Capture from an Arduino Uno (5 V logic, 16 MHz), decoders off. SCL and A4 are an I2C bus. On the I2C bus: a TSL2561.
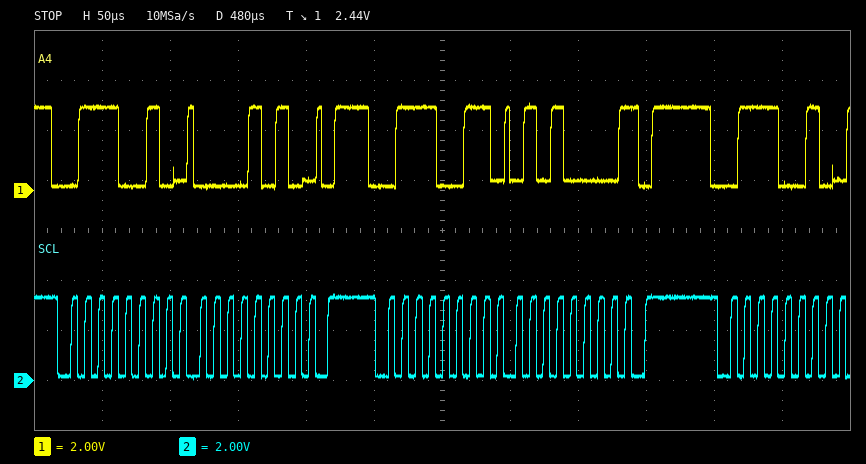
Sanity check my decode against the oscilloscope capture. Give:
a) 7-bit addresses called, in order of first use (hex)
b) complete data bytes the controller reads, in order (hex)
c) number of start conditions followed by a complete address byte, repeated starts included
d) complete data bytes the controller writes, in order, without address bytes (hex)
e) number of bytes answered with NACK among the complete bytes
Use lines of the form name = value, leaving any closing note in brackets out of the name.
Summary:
7-bit addresses called, in order of first use = 0x39
complete data bytes the controller reads, in order = 50
number of start conditions followed by a complete address byte, repeated starts included = 3
complete data bytes the controller writes, in order, without address bytes = 0A
number of bytes answered with NACK among the complete bytes = 1
